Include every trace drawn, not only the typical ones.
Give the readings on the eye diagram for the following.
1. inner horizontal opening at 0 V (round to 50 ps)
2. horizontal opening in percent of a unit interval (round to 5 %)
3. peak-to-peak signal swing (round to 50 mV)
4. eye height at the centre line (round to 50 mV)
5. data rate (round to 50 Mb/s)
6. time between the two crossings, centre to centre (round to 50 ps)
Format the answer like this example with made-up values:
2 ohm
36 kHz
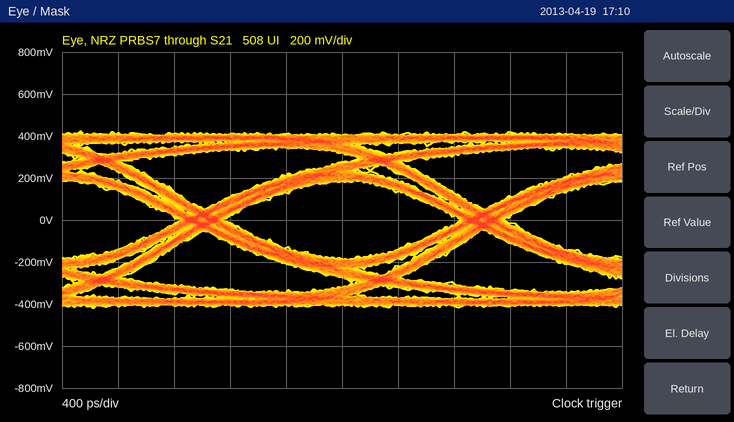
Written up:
1.70 ns
85 %
850 mV
350 mV
500 Mb/s
2.00 ns
